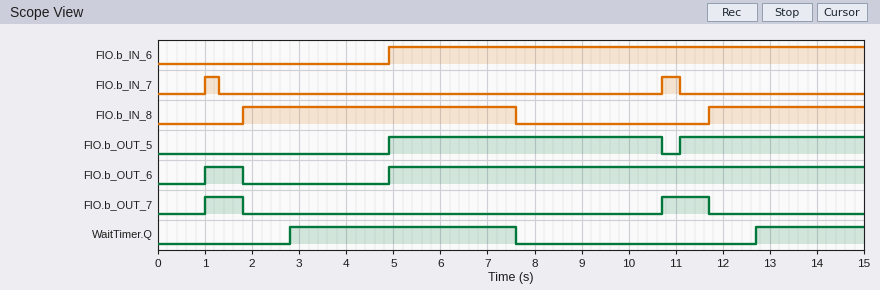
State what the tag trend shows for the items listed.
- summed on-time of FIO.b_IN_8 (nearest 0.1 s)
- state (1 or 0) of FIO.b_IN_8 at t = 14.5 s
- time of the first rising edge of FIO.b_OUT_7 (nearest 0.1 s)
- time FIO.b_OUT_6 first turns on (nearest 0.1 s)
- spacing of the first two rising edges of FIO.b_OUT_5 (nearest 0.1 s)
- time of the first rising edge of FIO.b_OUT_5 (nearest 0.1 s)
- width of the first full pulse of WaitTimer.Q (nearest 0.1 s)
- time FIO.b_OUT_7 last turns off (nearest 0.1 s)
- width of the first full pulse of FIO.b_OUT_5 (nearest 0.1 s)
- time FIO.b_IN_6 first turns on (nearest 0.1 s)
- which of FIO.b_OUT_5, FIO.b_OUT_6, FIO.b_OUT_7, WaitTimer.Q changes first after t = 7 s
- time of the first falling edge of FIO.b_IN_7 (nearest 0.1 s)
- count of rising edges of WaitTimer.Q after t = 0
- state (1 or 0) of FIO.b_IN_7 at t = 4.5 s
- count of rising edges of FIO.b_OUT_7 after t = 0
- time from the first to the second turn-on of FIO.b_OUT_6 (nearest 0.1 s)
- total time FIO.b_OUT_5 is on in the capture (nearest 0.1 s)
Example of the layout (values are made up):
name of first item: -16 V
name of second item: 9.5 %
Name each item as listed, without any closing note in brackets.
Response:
summed on-time of FIO.b_IN_8: 9.1 s
state (1 or 0) of FIO.b_IN_8 at t = 14.5 s: 1
time of the first rising edge of FIO.b_OUT_7: 1.0 s
time FIO.b_OUT_6 first turns on: 1.0 s
spacing of the first two rising edges of FIO.b_OUT_5: 6.2 s
time of the first rising edge of FIO.b_OUT_5: 4.9 s
width of the first full pulse of WaitTimer.Q: 4.8 s
time FIO.b_OUT_7 last turns off: 11.7 s
width of the first full pulse of FIO.b_OUT_5: 5.8 s
time FIO.b_IN_6 first turns on: 4.9 s
which of FIO.b_OUT_5, FIO.b_OUT_6, FIO.b_OUT_7, WaitTimer.Q changes first after t = 7 s: WaitTimer.Q
time of the first falling edge of FIO.b_IN_7: 1.3 s
count of rising edges of WaitTimer.Q after t = 0: 2
state (1 or 0) of FIO.b_IN_7 at t = 4.5 s: 0
count of rising edges of FIO.b_OUT_7 after t = 0: 2
time from the first to the second turn-on of FIO.b_OUT_6: 3.9 s
total time FIO.b_OUT_5 is on in the capture: 9.7 s
